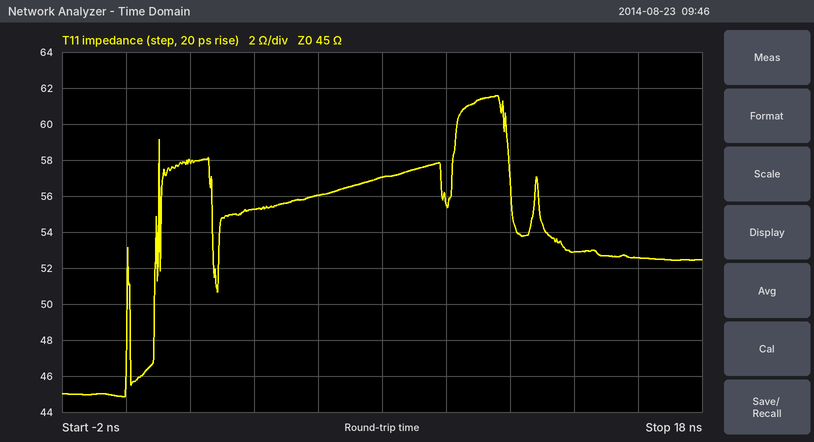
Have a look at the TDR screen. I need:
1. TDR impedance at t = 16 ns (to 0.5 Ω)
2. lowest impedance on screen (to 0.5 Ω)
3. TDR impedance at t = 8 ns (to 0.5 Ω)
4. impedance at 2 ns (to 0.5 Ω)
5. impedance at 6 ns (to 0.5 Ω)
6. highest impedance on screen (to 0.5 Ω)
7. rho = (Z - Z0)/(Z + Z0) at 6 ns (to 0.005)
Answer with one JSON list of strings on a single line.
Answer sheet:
["52.5 Ω", "45.0 Ω", "57.0 Ω", "58.0 Ω", "56.0 Ω", "61.5 Ω", "+0.110"]
